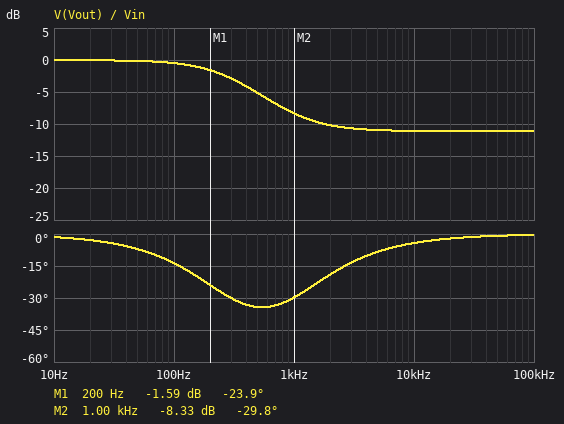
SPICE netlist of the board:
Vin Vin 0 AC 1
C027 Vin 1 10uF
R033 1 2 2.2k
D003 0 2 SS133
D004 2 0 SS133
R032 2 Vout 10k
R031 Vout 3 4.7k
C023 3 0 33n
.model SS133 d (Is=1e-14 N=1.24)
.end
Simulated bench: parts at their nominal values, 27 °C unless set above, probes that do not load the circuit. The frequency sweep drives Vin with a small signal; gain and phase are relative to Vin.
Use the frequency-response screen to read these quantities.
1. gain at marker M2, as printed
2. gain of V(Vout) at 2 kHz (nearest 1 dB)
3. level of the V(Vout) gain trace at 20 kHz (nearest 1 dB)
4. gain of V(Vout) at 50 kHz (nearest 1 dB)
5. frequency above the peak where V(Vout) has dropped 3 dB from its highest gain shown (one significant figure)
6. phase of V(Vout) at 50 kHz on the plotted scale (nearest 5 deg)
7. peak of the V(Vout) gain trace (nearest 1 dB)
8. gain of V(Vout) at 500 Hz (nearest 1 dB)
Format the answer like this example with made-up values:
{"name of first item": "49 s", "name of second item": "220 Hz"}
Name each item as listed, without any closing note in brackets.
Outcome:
{"gain at marker M2, as printed": "-8.33 dB", "gain of V(Vout) at 2 kHz": "-10 dB", "level of the V(Vout) gain trace at 20 kHz": "-11 dB", "gain of V(Vout) at 50 kHz": "-11 dB", "frequency above the peak where V(Vout) has dropped 3 dB from its highest gain shown": "300 Hz", "phase of V(Vout) at 50 kHz on the plotted scale": "0 deg", "peak of the V(Vout) gain trace": "0 dB", "gain of V(Vout) at 500 Hz": "-5 dB"}
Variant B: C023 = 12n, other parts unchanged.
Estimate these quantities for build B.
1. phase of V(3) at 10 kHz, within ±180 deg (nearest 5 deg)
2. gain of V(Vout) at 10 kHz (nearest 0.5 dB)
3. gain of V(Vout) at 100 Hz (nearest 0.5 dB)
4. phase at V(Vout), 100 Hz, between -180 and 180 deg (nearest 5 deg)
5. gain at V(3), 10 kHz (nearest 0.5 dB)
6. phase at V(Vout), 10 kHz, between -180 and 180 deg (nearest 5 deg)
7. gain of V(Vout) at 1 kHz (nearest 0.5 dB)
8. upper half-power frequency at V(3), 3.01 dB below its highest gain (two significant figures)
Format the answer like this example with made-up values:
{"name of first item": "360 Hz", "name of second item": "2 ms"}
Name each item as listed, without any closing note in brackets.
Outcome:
{"phase of V(3) at 10 kHz, within ±180 deg": "-85 deg", "gain of V(Vout) at 10 kHz": "-11.0 dB", "gain of V(Vout) at 100 Hz": "0 dB", "phase at V(Vout), 100 Hz, between -180 and 180 deg": "-5 deg", "gain at V(3), 10 kHz": "-22.0 dB", "phase at V(Vout), 10 kHz, between -180 and 180 deg": "-10 deg", "gain of V(Vout) at 1 kHz": "-3.5 dB", "upper half-power frequency at V(3), 3.01 dB below its highest gain": "790 Hz"}
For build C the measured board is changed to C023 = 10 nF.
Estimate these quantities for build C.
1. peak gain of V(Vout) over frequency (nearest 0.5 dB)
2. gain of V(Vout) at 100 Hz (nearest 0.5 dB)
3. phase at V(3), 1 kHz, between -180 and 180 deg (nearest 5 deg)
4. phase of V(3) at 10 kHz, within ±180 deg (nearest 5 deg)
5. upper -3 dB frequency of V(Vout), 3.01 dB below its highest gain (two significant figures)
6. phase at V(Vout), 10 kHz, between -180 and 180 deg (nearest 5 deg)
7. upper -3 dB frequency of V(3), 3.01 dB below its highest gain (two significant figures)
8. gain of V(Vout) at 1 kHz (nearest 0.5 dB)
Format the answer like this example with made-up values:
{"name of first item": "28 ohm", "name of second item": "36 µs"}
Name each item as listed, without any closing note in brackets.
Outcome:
{"peak gain of V(Vout) over frequency": "0 dB", "gain of V(Vout) at 100 Hz": "0 dB", "phase at V(3), 1 kHz, between -180 and 180 deg": "-45 deg", "phase of V(3) at 10 kHz, within ±180 deg": "-85 deg", "upper -3 dB frequency of V(Vout), 3.01 dB below its highest gain": "1.0 kHz", "phase at V(Vout), 10 kHz, between -180 and 180 deg": "-15 deg", "upper -3 dB frequency of V(3), 3.01 dB below its highest gain": "940 Hz", "gain of V(Vout) at 1 kHz": "-3.0 dB"}
